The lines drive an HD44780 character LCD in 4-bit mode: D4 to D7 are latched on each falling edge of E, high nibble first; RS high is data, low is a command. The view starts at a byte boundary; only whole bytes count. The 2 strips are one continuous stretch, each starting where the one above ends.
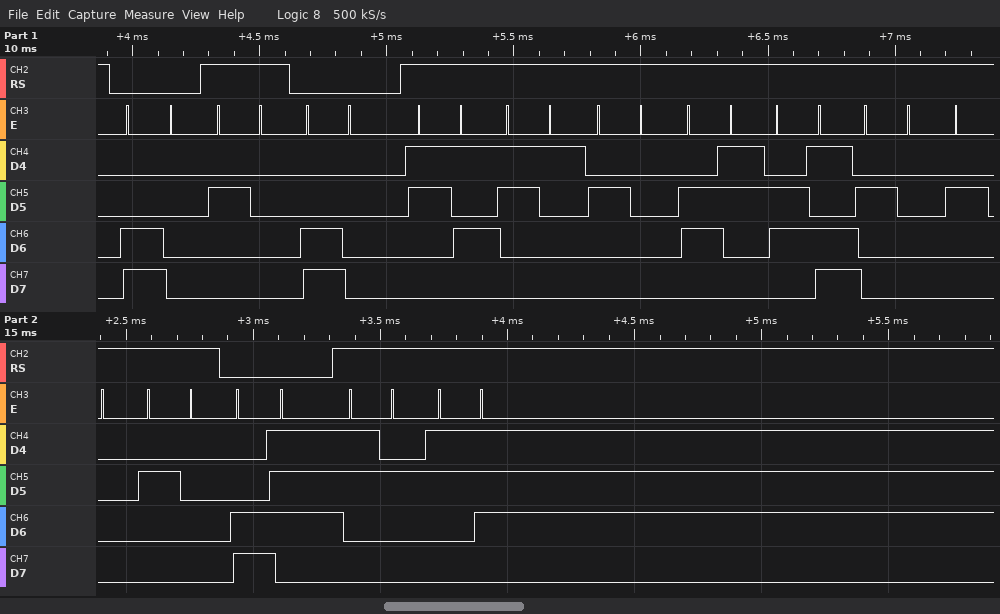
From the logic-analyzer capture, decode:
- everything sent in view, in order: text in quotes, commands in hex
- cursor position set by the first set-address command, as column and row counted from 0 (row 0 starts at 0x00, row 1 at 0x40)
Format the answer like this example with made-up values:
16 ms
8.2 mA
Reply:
0xC0 " " 0xC0 "51 cm   " 0xC7 "27"
column 0, row 1
